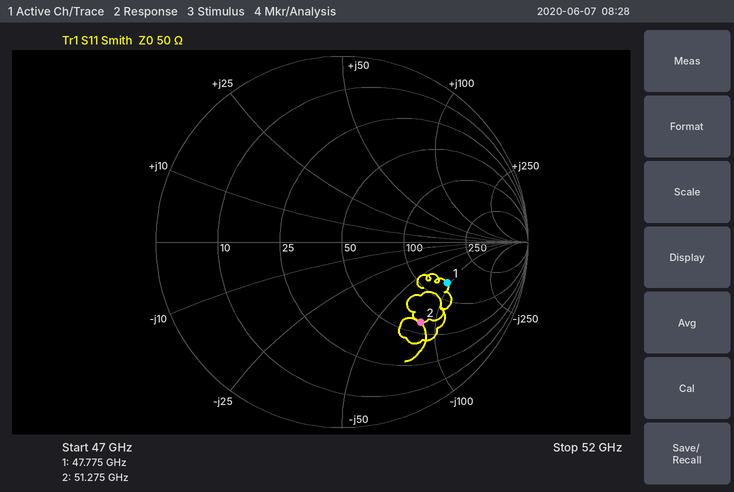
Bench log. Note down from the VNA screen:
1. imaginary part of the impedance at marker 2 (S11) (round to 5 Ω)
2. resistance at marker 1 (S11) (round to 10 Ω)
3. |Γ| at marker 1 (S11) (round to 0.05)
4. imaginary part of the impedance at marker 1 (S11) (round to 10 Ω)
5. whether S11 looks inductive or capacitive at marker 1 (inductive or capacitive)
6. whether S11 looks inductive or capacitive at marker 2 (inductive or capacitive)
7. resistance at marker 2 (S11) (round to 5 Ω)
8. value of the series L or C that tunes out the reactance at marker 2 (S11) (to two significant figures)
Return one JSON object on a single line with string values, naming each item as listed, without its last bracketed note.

{"imaginary part of the impedance at marker 2 (S11)": "-85 Ω", "resistance at marker 1 (S11)": "130 Ω", "|Γ| at marker 1 (S11)": "0.60", "imaginary part of the impedance at marker 1 (S11)": "-90 Ω", "whether S11 looks inductive or capacitive at marker 1": "capacitive", "whether S11 looks inductive or capacitive at marker 2": "capacitive", "resistance at marker 2 (S11)": "60 Ω", "value of the series L or C that tunes out the reactance at marker 2 (S11)": "260 pH"}
